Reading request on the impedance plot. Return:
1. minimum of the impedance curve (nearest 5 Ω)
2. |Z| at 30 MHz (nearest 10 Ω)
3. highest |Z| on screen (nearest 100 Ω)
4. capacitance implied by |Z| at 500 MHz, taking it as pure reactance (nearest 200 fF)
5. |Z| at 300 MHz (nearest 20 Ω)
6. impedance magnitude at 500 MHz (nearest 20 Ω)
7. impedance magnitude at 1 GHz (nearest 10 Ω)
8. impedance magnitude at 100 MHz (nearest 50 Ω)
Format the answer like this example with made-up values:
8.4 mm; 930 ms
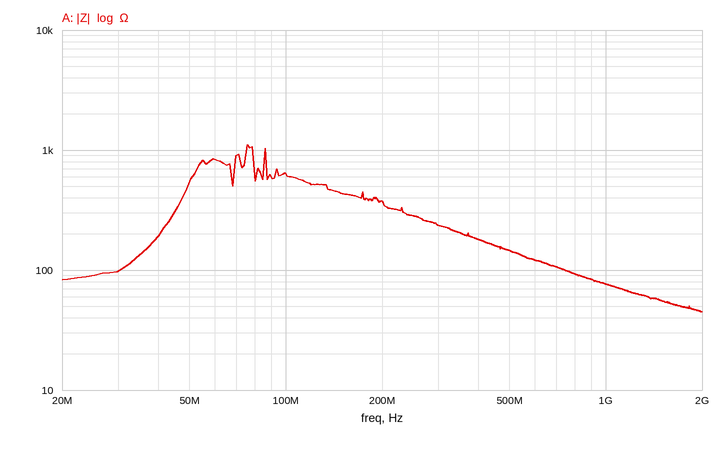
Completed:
45 Ω; 100 Ω; 1.1 kΩ; 2.2 pF; 240 Ω; 140 Ω; 80 Ω; 650 Ω
